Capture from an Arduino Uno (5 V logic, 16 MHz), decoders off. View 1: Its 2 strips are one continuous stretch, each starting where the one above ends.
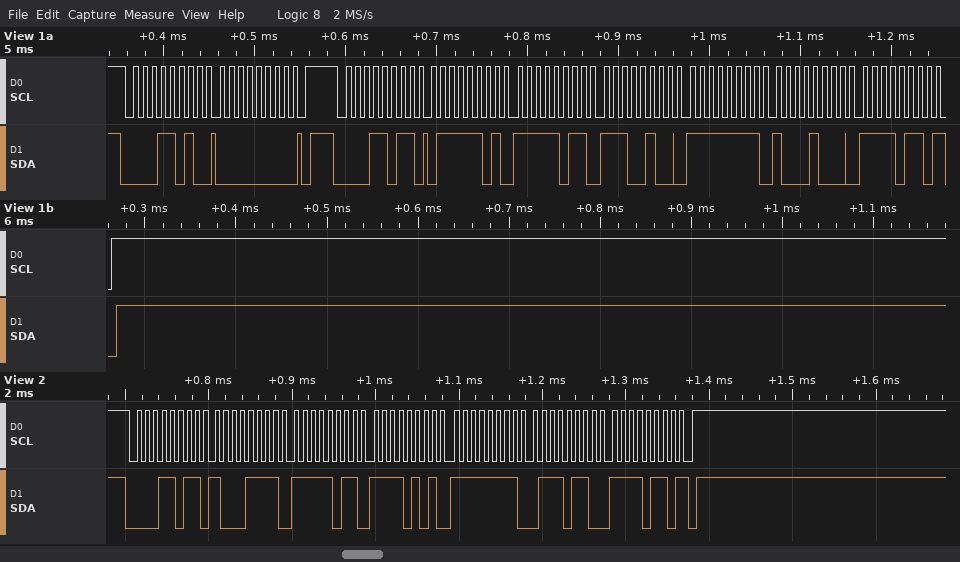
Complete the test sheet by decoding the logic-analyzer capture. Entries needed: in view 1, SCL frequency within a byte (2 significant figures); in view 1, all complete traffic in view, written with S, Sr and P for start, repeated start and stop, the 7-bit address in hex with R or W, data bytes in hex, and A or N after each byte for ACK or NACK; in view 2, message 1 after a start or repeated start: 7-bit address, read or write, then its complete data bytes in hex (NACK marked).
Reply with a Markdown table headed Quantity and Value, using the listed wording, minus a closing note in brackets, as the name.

| Quantity | Value |
|---|---|
| in view 1, SCL frequency within a byte | 100 kHz |
| in view 1, all complete traffic in view, written with S, Sr and P for start, repeated start and stop, the 7-bit address in hex with R or W, data bytes in hex, and A or N after each byte for ACK or NACK | S 0DW A 00 A P S 0DR A 7D A FB A E4 A FF A 88 A F6 N P |
| in view 2, message 1 after a start or repeated start: 7-bit address, read or write, then its complete data bytes in hex | 0x0D read: 8F FB F5 FF 76 F6 NACK |
